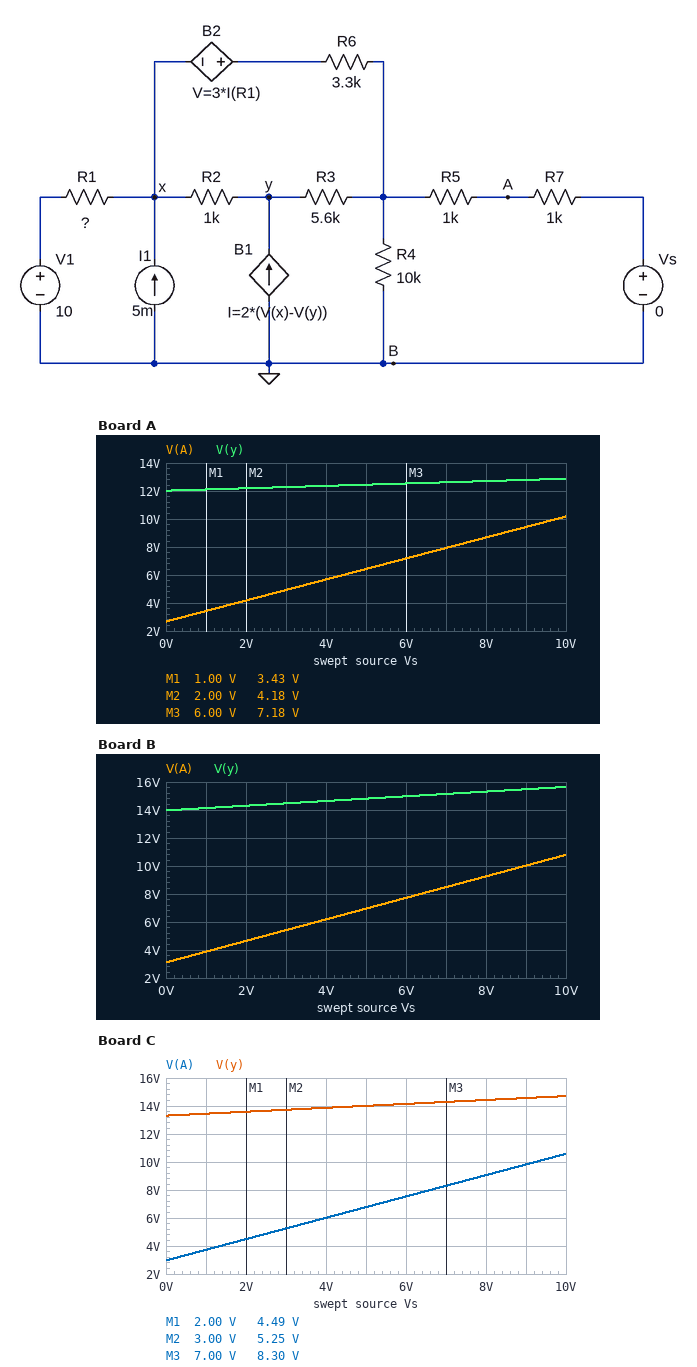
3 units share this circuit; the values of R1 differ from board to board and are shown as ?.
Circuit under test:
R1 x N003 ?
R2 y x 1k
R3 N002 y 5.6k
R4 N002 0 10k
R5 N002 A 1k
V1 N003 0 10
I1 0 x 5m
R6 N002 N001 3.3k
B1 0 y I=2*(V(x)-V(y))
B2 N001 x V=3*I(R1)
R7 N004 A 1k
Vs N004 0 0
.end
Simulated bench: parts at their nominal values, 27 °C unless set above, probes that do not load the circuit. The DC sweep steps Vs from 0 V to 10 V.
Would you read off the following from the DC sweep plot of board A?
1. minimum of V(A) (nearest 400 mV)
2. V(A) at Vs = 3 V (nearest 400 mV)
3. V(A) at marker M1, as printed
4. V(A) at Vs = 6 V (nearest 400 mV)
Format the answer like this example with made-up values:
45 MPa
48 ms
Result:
2.8 V
4.8 V
3.43 V
7.2 V
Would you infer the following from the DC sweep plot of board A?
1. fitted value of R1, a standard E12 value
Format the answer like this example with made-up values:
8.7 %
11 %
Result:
680 Ω
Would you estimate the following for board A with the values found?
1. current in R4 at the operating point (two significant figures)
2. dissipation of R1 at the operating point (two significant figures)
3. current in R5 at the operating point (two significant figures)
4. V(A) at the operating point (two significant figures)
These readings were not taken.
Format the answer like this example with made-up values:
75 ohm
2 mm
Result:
540 µA
6.0 mW
2.7 mA
2.7 V
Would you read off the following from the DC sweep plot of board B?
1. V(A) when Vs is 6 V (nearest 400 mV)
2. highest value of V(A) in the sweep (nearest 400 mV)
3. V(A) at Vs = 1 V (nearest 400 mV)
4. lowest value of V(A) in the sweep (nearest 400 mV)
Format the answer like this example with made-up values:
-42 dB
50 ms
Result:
7.6 V
10.8 V
4.0 V
3.2 V
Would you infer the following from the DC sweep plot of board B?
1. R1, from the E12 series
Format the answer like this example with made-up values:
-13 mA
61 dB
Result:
1.5 kΩ
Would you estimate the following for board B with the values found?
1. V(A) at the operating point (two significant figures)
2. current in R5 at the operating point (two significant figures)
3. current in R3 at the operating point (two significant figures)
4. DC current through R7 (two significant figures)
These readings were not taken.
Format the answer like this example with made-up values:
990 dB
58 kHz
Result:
3.1 V
3.1 mA
1.4 mA
3.1 mA
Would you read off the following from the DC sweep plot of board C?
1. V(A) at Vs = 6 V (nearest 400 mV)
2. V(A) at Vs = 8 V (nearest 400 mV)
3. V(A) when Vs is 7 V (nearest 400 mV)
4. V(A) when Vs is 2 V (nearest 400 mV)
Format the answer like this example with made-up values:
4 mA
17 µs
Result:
7.6 V
9.2 V
8.4 V
4.4 V
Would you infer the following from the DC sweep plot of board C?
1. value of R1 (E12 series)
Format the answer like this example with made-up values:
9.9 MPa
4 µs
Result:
1.2 kΩ
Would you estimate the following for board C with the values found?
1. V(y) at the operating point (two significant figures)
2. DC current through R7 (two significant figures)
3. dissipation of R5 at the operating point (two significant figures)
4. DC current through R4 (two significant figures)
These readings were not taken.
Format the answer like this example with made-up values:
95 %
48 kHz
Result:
13 V
3.0 mA
8.8 mW
590 µA
